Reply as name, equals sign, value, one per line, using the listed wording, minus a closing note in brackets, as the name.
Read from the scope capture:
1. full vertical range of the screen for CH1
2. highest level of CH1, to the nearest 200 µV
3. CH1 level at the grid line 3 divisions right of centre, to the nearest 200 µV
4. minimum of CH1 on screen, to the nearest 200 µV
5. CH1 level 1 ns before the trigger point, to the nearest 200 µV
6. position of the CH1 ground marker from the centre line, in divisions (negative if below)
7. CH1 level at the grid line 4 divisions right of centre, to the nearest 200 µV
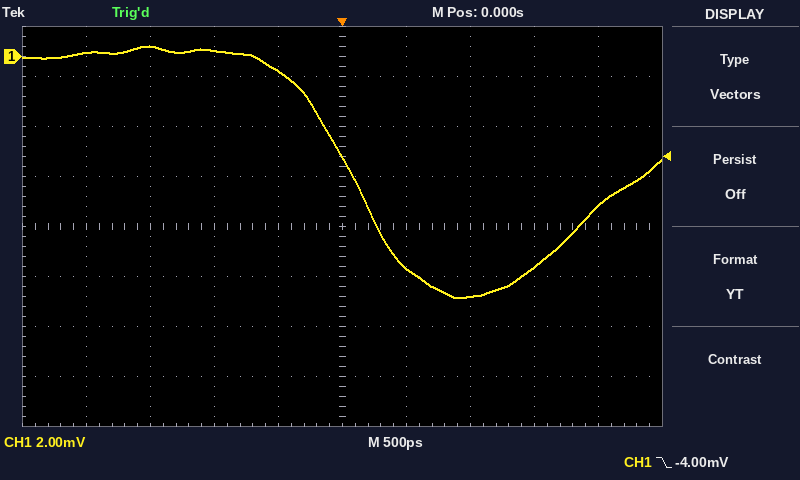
full vertical range of the screen for CH1 = 16 mV
highest level of CH1, to the nearest 200 µV = 400 µV
CH1 level at the grid line 3 divisions right of centre, to the nearest 200 µV = -8.4 mV
minimum of CH1 on screen, to the nearest 200 µV = -9.6 mV
CH1 level 1 ns before the trigger point, to the nearest 200 µV = 200 µV
position of the CH1 ground marker from the centre line, in divisions = +3.4 div
CH1 level at the grid line 4 divisions right of centre, to the nearest 200 µV = -6.0 mV
